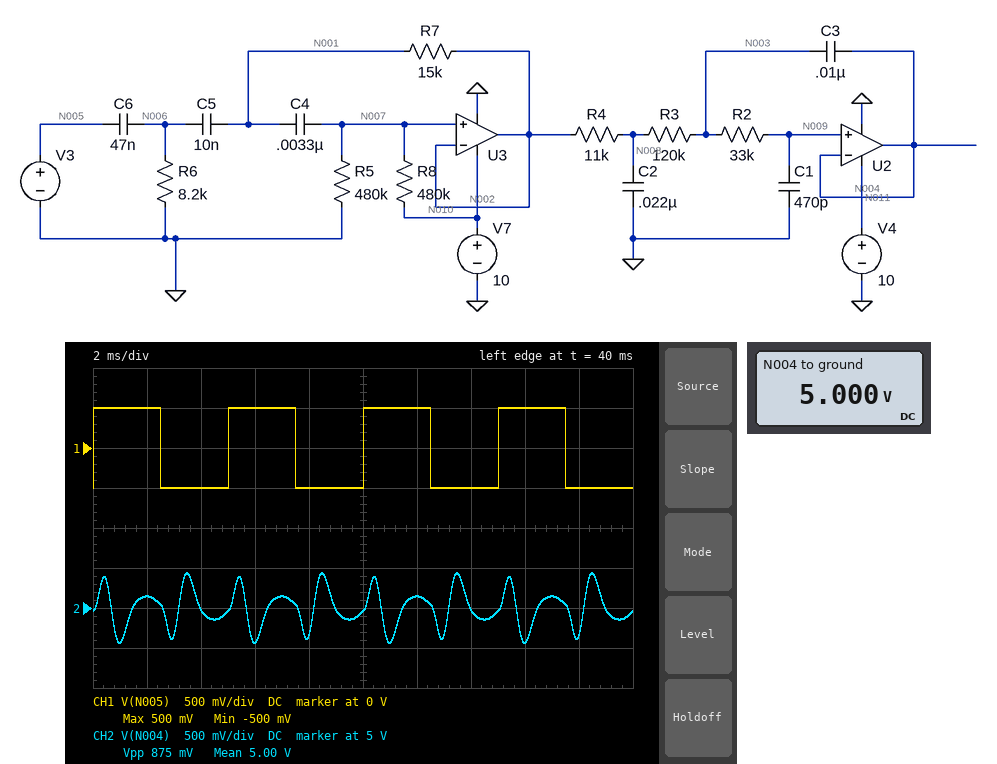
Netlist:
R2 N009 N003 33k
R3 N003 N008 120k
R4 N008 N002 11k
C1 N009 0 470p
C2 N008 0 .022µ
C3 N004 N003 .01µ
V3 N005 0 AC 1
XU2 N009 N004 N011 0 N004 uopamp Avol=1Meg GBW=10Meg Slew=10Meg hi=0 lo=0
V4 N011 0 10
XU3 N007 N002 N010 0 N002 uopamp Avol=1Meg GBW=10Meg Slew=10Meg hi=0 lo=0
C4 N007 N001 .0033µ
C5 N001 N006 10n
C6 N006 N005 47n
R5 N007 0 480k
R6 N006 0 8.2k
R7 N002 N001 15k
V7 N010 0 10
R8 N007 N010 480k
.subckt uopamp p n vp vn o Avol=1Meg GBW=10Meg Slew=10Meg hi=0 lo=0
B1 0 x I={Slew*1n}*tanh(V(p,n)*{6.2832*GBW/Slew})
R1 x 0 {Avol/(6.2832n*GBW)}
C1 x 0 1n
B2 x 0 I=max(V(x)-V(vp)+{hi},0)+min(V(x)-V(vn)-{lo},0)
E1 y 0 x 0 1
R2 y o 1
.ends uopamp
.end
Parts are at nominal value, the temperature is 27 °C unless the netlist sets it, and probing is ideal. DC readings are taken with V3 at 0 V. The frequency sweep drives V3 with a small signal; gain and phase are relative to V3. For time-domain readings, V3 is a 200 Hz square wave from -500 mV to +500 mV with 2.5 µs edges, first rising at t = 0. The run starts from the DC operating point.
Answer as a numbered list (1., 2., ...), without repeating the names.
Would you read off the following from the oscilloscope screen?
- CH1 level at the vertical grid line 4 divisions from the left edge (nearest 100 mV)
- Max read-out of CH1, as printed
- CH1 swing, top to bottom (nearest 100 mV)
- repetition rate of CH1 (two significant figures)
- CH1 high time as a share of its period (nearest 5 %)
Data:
1. -500 mV
2. 500 mV
3. 1.0 V
4. 200 Hz
5. 50 %
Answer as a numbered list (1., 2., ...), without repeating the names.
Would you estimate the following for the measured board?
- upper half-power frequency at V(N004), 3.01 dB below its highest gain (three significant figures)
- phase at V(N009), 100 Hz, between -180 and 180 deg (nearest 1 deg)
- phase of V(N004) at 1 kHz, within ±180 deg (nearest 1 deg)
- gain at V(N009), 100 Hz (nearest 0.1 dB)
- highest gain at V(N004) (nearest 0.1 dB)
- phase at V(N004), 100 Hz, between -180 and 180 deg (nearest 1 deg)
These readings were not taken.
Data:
1. 1.20 kHz
2. -125 deg
3. -75 deg
4. -39.0 dB
5. 1.9 dB
6. -125 deg
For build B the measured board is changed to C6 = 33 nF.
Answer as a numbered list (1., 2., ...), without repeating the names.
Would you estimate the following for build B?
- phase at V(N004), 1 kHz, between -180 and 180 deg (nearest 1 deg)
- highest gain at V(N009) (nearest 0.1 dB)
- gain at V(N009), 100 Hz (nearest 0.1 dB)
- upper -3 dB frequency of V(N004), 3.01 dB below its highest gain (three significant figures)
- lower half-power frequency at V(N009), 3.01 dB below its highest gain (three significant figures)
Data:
1. -66 deg
2. 0.6 dB
3. -41.9 dB
4. 1.25 kHz
5. 456 Hz
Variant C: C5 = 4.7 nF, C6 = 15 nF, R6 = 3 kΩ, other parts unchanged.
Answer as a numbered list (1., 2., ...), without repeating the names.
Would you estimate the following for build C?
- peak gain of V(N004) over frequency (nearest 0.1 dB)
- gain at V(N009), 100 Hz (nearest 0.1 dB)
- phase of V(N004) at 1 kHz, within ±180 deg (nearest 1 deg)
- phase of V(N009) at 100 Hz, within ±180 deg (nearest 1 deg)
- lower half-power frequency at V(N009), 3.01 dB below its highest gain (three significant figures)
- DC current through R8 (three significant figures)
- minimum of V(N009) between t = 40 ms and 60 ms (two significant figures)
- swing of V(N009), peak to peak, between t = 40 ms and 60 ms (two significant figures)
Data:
1. -7.9 dB
2. -64.0 dB
3. -10 deg
4. -108 deg
5. 648 Hz
6. 10.4 µA
7. 4.9 V
8. 240 mV
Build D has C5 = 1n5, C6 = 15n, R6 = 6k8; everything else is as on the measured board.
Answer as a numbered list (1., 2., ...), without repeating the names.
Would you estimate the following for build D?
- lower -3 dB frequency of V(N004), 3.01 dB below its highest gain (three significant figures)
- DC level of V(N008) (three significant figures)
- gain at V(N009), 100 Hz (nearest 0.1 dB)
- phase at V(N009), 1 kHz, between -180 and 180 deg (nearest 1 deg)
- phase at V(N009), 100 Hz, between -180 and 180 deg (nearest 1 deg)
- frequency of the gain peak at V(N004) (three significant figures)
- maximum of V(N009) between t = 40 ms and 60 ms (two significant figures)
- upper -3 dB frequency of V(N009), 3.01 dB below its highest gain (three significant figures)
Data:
1. 976 Hz
2. 5.00 V
3. -66.9 dB
4. 60 deg
5. -108 deg
6. 1.18 kHz
7. 5.2 V
8. 1.41 kHz
